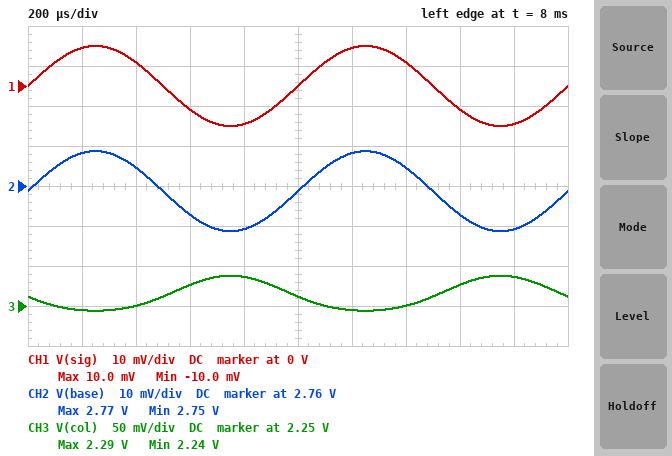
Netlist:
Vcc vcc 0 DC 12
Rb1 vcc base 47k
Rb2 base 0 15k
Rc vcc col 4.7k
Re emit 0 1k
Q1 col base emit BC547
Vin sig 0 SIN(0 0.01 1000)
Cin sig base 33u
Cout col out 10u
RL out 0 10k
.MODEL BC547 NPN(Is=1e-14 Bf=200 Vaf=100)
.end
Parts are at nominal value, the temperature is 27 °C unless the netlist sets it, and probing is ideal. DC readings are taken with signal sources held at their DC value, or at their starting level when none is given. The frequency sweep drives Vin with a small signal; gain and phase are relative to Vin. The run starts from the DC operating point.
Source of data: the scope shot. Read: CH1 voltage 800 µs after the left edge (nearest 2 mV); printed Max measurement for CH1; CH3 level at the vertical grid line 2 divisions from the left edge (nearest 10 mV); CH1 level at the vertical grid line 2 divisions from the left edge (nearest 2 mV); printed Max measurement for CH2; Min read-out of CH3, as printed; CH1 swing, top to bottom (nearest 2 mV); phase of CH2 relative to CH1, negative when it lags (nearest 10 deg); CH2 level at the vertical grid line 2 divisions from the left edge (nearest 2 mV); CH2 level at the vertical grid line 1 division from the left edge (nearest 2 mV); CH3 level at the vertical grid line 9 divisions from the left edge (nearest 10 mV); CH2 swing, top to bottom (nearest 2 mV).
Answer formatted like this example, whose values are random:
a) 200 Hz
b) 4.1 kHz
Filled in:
a) -10 mV
b) 10.0 mV
c) 2.25 V
d) 6 mV
e) 2.77 V
f) 2.24 V
g) 20 mV
h) 0 deg
i) 2.764 V
j) 2.768 V
k) 2.29 V
l) 20 mV
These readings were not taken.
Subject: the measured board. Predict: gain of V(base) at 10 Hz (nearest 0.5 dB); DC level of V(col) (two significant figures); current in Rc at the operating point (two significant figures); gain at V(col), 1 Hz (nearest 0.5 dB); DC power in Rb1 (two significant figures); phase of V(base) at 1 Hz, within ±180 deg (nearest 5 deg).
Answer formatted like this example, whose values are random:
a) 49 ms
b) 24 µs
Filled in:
a) 0 dB
b) 2.3 V
c) 2.1 mA
d) 2.0 dB
e) 1.8 mW
f) 65 deg
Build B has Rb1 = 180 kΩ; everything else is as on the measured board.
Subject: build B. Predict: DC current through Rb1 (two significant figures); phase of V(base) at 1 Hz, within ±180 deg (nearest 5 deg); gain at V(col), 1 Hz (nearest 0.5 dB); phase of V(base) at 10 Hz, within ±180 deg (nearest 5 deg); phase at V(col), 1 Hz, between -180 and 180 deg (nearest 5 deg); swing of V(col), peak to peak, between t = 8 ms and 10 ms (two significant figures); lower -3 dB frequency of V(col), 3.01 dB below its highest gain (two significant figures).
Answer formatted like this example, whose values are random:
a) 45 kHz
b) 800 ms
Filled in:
a) 62 µA
b) 20 deg
c) 11.0 dB
d) 0 deg
e) -170 deg
f) 58 mV
g) 270 mHz
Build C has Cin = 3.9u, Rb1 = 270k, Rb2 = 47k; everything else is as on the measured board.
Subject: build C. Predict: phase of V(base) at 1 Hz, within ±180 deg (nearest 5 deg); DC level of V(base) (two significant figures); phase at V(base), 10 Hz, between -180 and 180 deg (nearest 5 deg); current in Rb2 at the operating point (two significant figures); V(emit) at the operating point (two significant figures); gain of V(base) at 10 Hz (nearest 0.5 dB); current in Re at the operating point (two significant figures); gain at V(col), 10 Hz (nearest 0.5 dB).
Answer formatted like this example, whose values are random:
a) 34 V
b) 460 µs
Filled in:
a) 50 deg
b) 1.6 V
c) 5 deg
d) 34 µA
e) 950 mV
f) 0 dB
g) 950 µA
h) 10.0 dB
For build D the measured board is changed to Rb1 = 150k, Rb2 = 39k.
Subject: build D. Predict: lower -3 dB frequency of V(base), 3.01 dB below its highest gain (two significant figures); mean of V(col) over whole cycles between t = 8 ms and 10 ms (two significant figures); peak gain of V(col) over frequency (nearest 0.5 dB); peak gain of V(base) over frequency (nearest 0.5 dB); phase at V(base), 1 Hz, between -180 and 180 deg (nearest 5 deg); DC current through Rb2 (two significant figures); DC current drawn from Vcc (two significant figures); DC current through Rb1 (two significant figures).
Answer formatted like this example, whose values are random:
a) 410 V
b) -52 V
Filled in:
a) 180 mHz
b) 4.6 V
c) 12.5 dB
d) 0 dB
e) 10 deg
f) 57 µA
g) 1.6 mA
h) 65 µA
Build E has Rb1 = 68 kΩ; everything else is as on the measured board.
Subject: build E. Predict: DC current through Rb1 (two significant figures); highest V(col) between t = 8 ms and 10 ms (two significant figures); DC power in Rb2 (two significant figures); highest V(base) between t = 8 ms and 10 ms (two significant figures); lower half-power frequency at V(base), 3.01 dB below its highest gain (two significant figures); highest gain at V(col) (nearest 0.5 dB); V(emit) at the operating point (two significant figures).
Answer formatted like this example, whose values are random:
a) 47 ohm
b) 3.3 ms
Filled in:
a) 150 µA
b) 5.4 V
c) 290 µW
d) 2.1 V
e) 420 mHz
f) 11.5 dB
g) 1.4 V
